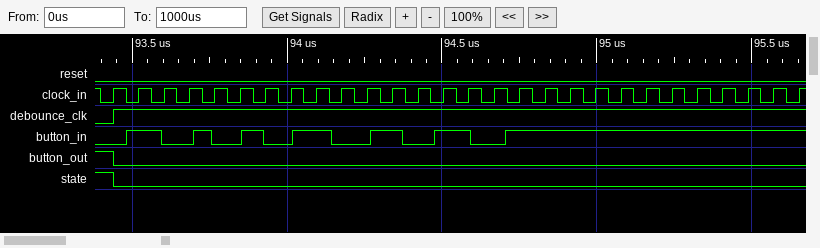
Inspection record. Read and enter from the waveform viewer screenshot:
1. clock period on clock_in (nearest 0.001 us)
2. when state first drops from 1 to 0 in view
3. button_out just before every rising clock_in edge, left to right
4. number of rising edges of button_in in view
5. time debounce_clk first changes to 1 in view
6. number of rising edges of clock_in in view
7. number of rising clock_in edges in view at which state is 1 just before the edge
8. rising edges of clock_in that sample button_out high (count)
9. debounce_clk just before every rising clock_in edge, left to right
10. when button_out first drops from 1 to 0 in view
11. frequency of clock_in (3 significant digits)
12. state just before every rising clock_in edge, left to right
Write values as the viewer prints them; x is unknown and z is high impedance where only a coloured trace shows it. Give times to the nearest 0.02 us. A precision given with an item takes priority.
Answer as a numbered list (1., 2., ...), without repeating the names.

1. 0.082 us
2. 93.44 us
3. 1 0 0 0 0 0 0 0 0 0 0 0 0 0 0 0 0 0 0 0 0 0 0 0 0 0 0 0
4. 7
5. 93.44 us
6. 28
7. 1
8. 1
9. 0 1 1 1 1 1 1 1 1 1 1 1 1 1 1 1 1 1 1 1 1 1 1 1 1 1 1 1
10. 93.44 us
11. 12.2 MHz
12. 1 0 0 0 0 0 0 0 0 0 0 0 0 0 0 0 0 0 0 0 0 0 0 0 0 0 0 0
